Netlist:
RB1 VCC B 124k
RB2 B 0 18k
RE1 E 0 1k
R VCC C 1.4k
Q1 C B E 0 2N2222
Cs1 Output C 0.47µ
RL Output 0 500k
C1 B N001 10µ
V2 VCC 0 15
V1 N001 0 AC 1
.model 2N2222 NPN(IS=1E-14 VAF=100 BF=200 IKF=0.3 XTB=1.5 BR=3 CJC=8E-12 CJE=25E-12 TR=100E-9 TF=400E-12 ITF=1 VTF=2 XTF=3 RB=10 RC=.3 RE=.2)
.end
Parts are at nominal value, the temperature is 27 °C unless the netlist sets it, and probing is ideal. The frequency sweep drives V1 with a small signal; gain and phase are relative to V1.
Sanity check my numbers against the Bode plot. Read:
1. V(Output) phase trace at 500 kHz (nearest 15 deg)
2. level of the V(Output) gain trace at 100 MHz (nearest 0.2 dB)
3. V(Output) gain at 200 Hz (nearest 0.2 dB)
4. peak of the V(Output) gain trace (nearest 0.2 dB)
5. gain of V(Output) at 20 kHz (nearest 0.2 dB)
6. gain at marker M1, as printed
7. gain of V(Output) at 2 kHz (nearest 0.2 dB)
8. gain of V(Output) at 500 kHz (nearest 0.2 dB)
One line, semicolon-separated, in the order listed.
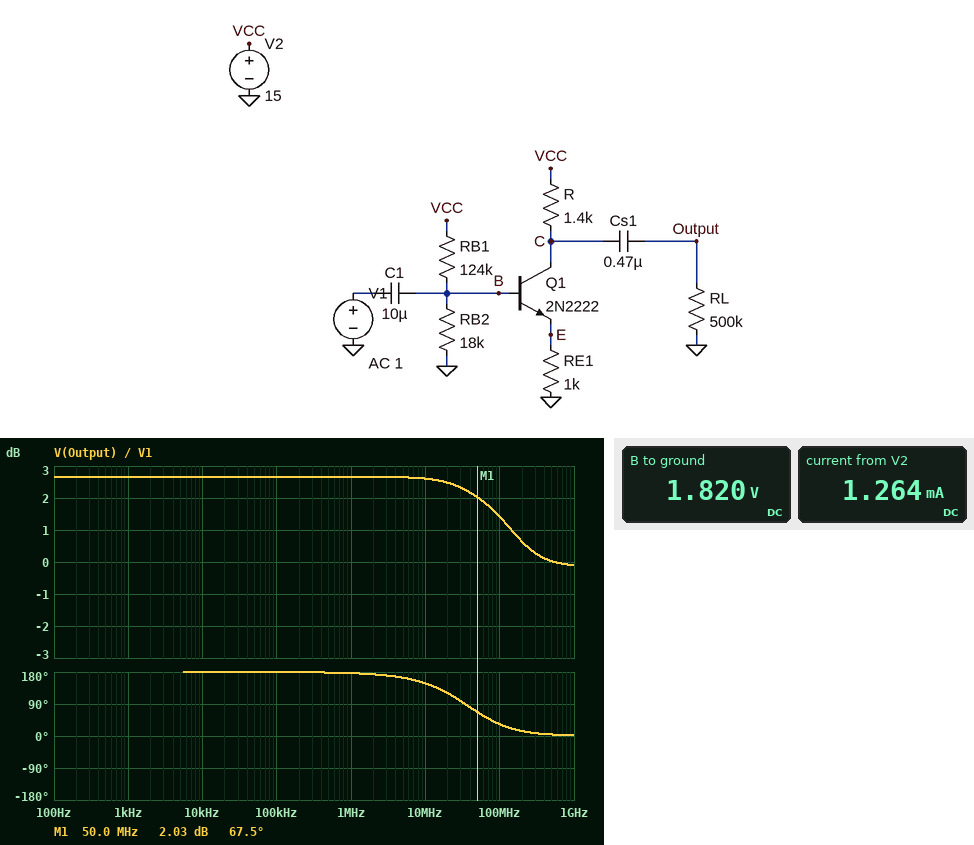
180 deg; 1.4 dB; 2.6 dB; 2.6 dB; 2.6 dB; 2.03 dB; 2.6 dB; 2.6 dB
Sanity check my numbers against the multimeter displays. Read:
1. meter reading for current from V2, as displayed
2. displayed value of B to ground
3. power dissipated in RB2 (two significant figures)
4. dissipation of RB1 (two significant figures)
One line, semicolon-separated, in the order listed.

1.264 mA; 1.820 V; 180 µW; 1.4 mW
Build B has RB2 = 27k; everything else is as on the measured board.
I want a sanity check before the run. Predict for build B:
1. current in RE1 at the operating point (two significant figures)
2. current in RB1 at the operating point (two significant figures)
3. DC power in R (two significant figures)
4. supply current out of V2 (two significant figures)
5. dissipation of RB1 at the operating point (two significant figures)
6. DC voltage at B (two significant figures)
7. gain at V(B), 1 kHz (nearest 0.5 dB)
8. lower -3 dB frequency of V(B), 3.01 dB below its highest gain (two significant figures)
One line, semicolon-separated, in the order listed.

1.8 mA; 100 µA; 4.6 mW; 1.9 mA; 1.3 mW; 2.5 V; 0 dB; 790 mHz
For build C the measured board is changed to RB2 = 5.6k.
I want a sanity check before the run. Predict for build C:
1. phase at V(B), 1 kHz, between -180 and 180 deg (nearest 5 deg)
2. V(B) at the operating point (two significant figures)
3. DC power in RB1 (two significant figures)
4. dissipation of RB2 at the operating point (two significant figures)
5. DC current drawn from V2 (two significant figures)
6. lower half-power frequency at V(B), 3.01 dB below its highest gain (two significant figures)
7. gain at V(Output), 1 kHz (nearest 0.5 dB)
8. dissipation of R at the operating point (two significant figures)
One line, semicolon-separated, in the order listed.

0 deg; 650 mV; 1.7 mW; 75 µW; 180 µA; 3.0 Hz; 0 dB; 6.0 µW
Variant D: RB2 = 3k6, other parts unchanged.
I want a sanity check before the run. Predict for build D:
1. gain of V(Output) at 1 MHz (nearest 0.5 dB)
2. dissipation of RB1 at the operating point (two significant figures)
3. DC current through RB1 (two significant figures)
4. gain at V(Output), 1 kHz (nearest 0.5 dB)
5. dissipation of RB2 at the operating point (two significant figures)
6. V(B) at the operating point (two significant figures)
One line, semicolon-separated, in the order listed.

-31.0 dB; 1.7 mW; 120 µA; -42.0 dB; 50 µW; 420 mV
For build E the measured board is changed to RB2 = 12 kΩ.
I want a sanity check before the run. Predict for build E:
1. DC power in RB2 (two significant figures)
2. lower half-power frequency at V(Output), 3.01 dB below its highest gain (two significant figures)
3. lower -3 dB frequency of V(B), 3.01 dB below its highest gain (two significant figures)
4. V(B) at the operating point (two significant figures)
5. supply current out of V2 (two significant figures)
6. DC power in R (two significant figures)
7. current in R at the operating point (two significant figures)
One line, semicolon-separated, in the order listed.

140 µW; 1.8 Hz; 1.5 Hz; 1.3 V; 760 µA; 590 µW; 650 µA
